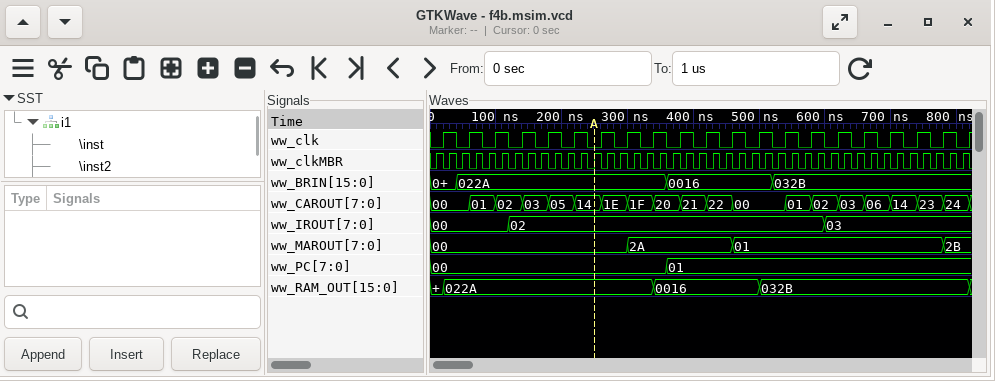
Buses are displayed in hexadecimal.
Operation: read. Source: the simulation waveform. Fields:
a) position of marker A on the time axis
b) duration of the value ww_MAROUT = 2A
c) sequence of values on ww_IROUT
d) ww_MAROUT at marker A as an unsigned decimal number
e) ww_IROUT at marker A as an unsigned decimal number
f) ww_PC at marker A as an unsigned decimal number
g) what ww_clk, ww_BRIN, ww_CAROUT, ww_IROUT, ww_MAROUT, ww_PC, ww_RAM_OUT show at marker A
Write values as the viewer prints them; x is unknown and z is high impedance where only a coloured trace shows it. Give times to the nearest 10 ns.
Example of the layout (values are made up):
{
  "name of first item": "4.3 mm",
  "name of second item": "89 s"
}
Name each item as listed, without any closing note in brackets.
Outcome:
{
  "position of marker A on the time axis": "250 ns",
  "duration of the value ww_MAROUT = 2A": "160 ns",
  "sequence of values on ww_IROUT": "00, 02, 03",
  "ww_MAROUT at marker A as an unsigned decimal number": "0",
  "ww_IROUT at marker A as an unsigned decimal number": "2",
  "ww_PC at marker A as an unsigned decimal number": "0",
  "what ww_clk, ww_BRIN, ww_CAROUT, ww_IROUT, ww_MAROUT, ww_PC, ww_RAM_OUT show at marker A": "ww_clk=0, ww_BRIN=022A, ww_CAROUT=14, ww_IROUT=02, ww_MAROUT=00, ww_PC=00, ww_RAM_OUT=022A"
}
